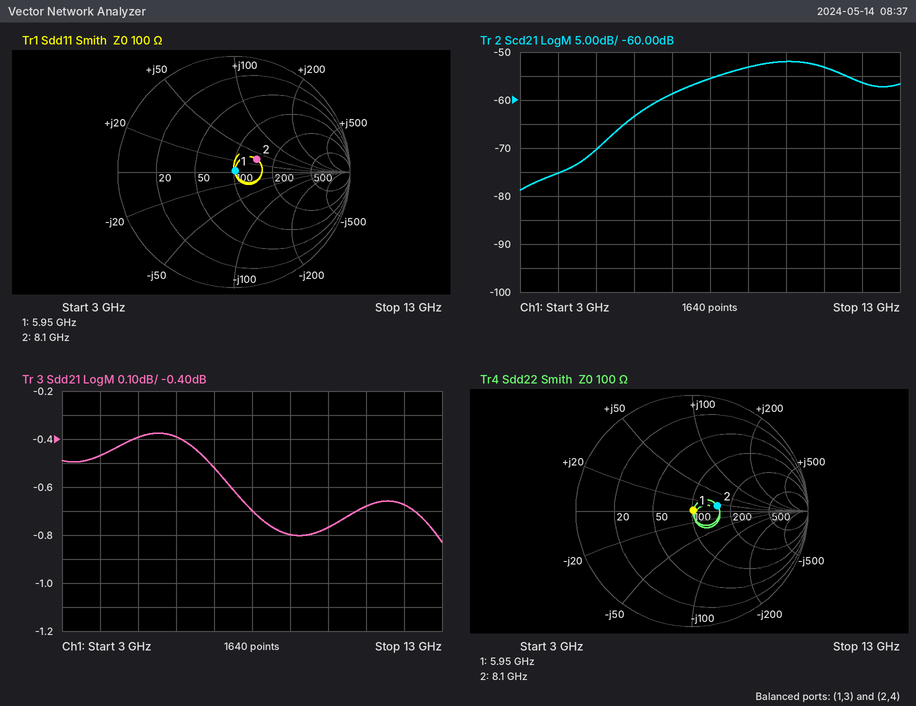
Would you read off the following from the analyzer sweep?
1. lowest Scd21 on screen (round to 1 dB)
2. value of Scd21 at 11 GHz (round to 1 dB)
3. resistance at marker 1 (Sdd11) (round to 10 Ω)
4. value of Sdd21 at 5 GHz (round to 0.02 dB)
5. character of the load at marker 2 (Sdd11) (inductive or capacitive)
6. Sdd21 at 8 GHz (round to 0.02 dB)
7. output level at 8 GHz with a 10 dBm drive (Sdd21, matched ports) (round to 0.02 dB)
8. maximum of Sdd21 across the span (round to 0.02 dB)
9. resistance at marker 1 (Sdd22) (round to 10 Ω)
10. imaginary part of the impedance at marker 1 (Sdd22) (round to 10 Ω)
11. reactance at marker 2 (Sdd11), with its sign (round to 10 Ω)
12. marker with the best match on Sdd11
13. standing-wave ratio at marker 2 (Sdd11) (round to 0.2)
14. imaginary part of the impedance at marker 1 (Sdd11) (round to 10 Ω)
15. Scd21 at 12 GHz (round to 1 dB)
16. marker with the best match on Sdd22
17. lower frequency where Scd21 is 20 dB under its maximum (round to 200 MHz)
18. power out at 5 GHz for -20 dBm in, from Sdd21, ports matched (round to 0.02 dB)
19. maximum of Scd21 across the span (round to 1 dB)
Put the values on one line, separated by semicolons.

-79 dB; -53 dB; 100 Ω; -0.40 dB; inductive; -0.70 dB; 9.30 dBm; -0.38 dB; 100 Ω; 0 Ω; +30 Ω; marker 1; 1.6; 0 Ω; -56 dB; marker 1; 4.8 GHz; -20.40 dBm; -52 dB
